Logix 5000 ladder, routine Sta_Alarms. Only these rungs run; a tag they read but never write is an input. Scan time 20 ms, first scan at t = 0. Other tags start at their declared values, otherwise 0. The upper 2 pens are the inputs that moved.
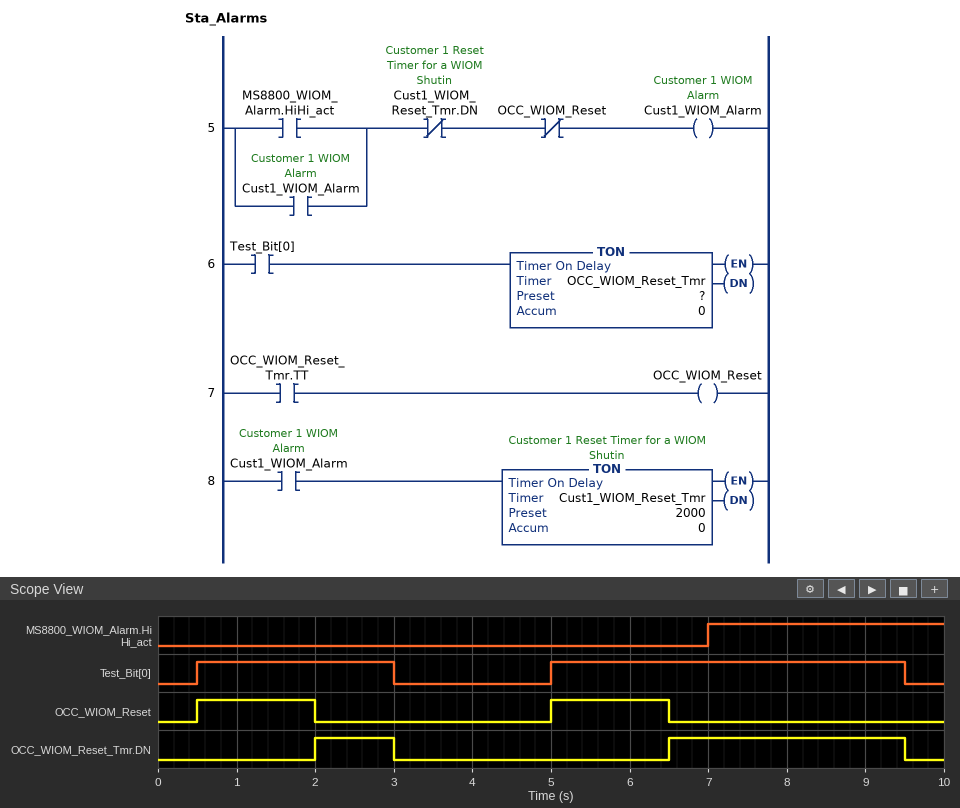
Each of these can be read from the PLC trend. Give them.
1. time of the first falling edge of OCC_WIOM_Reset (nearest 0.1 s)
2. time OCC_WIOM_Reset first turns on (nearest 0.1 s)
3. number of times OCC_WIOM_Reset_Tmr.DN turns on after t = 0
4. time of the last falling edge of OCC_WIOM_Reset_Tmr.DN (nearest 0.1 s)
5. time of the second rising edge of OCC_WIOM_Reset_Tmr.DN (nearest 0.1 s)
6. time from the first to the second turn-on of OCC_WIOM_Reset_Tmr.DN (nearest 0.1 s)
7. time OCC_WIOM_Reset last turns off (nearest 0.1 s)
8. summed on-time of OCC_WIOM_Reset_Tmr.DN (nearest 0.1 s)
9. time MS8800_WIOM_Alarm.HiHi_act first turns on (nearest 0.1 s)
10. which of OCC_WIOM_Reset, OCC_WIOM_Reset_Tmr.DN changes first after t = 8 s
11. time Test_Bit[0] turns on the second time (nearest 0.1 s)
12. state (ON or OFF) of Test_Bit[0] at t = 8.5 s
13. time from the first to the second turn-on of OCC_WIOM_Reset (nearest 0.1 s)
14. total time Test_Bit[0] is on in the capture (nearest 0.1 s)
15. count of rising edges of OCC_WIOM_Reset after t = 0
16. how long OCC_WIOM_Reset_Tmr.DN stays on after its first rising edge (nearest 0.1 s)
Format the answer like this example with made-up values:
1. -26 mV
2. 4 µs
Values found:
1. 2.0 s
2. 0.5 s
3. 2
4. 9.5 s
5. 6.5 s
6. 4.5 s
7. 6.5 s
8. 4.0 s
9. 7.0 s
10. OCC_WIOM_Reset_Tmr.DN
11. 5.0 s
12. ON
13. 4.5 s
14. 7.0 s
15. 2
16. 1.0 s
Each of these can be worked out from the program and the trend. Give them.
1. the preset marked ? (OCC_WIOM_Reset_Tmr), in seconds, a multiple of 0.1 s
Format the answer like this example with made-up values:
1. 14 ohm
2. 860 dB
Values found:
1. 1.5 s
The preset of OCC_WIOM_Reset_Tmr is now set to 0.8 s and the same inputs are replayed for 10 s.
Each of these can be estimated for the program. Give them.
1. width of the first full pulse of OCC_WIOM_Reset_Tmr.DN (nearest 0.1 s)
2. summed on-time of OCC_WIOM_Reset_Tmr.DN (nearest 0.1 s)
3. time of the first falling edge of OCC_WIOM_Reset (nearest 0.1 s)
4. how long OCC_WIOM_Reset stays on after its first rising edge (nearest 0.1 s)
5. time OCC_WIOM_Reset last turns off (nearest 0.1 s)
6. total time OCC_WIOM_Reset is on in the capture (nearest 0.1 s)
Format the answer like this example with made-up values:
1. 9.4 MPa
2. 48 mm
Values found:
1. 1.7 s
2. 5.4 s
3. 1.3 s
4. 0.8 s
5. 5.8 s
6. 1.6 s
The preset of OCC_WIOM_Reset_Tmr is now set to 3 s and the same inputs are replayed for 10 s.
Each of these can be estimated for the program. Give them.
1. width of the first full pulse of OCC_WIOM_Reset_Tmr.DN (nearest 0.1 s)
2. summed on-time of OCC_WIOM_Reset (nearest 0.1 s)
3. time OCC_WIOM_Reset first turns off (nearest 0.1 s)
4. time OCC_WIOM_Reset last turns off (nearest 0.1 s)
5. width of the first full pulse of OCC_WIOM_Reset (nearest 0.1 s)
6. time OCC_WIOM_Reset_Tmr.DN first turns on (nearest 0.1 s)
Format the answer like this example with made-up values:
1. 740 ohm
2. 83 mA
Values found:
1. 1.5 s
2. 5.5 s
3. 3.0 s
4. 8.0 s
5. 2.5 s
6. 8.0 s
